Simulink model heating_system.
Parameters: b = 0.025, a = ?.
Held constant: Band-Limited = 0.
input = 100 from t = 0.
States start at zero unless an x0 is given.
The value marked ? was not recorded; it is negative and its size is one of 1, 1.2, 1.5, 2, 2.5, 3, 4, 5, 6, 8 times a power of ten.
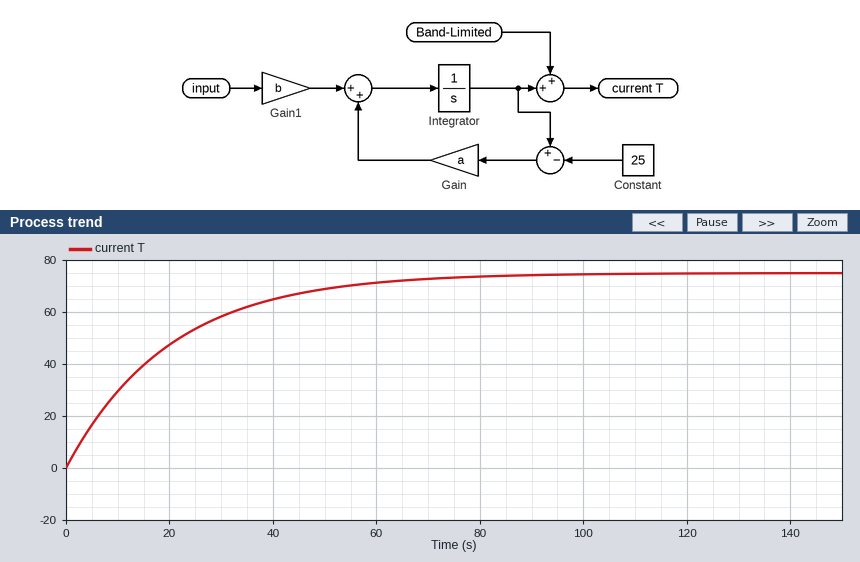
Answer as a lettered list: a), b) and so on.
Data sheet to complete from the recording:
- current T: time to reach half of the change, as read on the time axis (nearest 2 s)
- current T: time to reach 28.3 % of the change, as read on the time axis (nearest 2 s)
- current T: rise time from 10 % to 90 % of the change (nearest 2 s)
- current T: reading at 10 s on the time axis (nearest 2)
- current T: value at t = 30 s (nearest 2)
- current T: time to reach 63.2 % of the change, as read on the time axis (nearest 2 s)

a) 14 s
b) 6 s
c) 44 s
d) 30
e) 58
f) 20 s
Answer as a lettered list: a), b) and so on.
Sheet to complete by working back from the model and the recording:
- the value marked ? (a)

a) -0.05
